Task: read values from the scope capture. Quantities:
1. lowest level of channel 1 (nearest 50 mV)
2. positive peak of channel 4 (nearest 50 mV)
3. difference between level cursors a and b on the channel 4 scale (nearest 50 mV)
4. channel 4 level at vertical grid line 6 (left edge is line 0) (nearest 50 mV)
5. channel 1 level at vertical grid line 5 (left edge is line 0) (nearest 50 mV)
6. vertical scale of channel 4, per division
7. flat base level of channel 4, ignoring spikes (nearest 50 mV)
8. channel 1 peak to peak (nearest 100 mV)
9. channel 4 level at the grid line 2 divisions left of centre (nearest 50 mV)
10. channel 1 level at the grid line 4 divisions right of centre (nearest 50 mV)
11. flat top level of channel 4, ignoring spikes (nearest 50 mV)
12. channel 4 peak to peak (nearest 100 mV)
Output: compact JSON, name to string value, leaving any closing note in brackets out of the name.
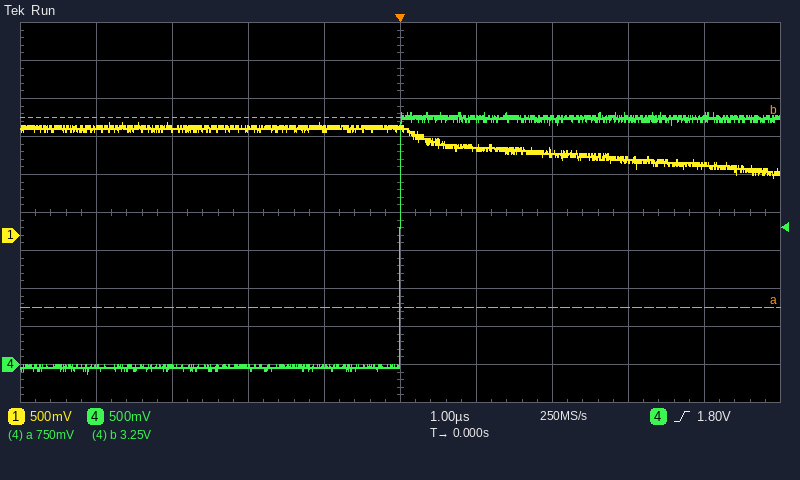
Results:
{"lowest level of channel 1": "750 mV", "positive peak of channel 4": "3.30 V", "difference between level cursors a and b on the channel 4 scale": "2.50 V", "channel 4 level at vertical grid line 6 (left edge is line 0)": "3.25 V", "channel 1 level at vertical grid line 5 (left edge is line 0)": "1.40 V", "vertical scale of channel 4, per division": "500 mV", "flat base level of channel 4, ignoring spikes": "-50 mV", "channel 1 peak to peak": "700 mV", "channel 4 level at the grid line 2 divisions left of centre": "-50 mV", "channel 1 level at the grid line 4 divisions right of centre": "900 mV", "flat top level of channel 4, ignoring spikes": "3.25 V", "channel 4 peak to peak": "3.40 V"}
